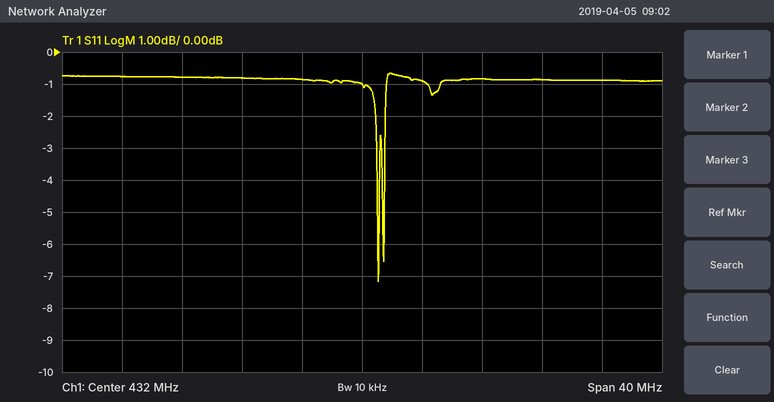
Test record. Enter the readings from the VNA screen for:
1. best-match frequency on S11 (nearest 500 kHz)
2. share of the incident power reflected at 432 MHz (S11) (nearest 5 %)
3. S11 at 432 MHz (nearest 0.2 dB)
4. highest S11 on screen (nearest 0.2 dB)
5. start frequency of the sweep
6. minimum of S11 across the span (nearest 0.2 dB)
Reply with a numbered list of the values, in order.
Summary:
1. 433.0 MHz
2. 80 %
3. -1.0 dB
4. -0.6 dB
5. 412 MHz
6. -7.2 dB
